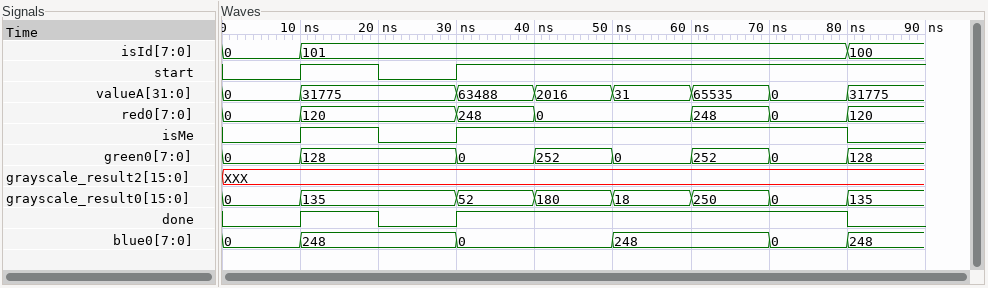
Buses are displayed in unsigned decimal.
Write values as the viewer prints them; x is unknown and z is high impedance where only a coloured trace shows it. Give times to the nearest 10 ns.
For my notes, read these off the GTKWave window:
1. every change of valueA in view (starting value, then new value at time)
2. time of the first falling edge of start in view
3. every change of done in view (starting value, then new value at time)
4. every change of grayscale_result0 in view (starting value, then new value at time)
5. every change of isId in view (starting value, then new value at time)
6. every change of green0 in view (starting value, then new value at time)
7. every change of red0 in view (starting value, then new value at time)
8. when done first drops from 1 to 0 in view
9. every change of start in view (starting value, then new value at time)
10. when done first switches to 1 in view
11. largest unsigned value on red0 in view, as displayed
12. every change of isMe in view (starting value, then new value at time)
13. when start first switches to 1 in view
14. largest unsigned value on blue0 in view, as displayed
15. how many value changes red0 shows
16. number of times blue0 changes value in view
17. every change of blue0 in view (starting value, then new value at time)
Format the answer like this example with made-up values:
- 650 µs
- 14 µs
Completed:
- 0, 31775 at 10 ns, 63488 at 30 ns, 2016 at 40 ns, 31 at 50 ns, 65535 at 60 ns, 0 at 70 ns, 31775 at 80 ns
- 20 ns
- 0, 1 at 10 ns, 0 at 20 ns, 1 at 30 ns, 0 at 80 ns
- 0, 135 at 10 ns, 52 at 30 ns, 180 at 40 ns, 18 at 50 ns, 250 at 60 ns, 0 at 70 ns, 135 at 80 ns
- 0, 101 at 10 ns, 100 at 80 ns
- 0, 128 at 10 ns, 0 at 30 ns, 252 at 40 ns, 0 at 50 ns, 252 at 60 ns, 0 at 70 ns, 128 at 80 ns
- 0, 120 at 10 ns, 248 at 30 ns, 0 at 40 ns, 248 at 60 ns, 0 at 70 ns, 120 at 80 ns
- 20 ns
- 0, 1 at 10 ns, 0 at 20 ns, 1 at 30 ns
- 10 ns
- 248
- 0, 1 at 10 ns, 0 at 20 ns, 1 at 30 ns, 0 at 80 ns
- 10 ns
- 248
- 6
- 5
- 0, 248 at 10 ns, 0 at 30 ns, 248 at 50 ns, 0 at 70 ns, 248 at 80 ns
